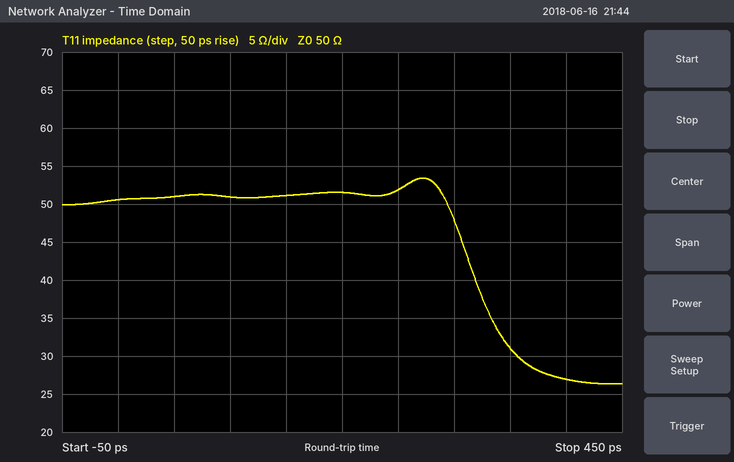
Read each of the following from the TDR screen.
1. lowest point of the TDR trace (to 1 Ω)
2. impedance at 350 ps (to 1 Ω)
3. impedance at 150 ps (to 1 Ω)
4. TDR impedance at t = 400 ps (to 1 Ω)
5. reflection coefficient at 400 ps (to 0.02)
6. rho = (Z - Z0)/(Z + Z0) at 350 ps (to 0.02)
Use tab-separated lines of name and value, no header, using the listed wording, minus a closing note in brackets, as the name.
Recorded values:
lowest point of the TDR trace	26 Ω
impedance at 350 ps	31 Ω
impedance at 150 ps	51 Ω
TDR impedance at t = 400 ps	27 Ω
reflection coefficient at 400 ps	-0.30
rho = (Z - Z0)/(Z + Z0) at 350 ps	-0.24
